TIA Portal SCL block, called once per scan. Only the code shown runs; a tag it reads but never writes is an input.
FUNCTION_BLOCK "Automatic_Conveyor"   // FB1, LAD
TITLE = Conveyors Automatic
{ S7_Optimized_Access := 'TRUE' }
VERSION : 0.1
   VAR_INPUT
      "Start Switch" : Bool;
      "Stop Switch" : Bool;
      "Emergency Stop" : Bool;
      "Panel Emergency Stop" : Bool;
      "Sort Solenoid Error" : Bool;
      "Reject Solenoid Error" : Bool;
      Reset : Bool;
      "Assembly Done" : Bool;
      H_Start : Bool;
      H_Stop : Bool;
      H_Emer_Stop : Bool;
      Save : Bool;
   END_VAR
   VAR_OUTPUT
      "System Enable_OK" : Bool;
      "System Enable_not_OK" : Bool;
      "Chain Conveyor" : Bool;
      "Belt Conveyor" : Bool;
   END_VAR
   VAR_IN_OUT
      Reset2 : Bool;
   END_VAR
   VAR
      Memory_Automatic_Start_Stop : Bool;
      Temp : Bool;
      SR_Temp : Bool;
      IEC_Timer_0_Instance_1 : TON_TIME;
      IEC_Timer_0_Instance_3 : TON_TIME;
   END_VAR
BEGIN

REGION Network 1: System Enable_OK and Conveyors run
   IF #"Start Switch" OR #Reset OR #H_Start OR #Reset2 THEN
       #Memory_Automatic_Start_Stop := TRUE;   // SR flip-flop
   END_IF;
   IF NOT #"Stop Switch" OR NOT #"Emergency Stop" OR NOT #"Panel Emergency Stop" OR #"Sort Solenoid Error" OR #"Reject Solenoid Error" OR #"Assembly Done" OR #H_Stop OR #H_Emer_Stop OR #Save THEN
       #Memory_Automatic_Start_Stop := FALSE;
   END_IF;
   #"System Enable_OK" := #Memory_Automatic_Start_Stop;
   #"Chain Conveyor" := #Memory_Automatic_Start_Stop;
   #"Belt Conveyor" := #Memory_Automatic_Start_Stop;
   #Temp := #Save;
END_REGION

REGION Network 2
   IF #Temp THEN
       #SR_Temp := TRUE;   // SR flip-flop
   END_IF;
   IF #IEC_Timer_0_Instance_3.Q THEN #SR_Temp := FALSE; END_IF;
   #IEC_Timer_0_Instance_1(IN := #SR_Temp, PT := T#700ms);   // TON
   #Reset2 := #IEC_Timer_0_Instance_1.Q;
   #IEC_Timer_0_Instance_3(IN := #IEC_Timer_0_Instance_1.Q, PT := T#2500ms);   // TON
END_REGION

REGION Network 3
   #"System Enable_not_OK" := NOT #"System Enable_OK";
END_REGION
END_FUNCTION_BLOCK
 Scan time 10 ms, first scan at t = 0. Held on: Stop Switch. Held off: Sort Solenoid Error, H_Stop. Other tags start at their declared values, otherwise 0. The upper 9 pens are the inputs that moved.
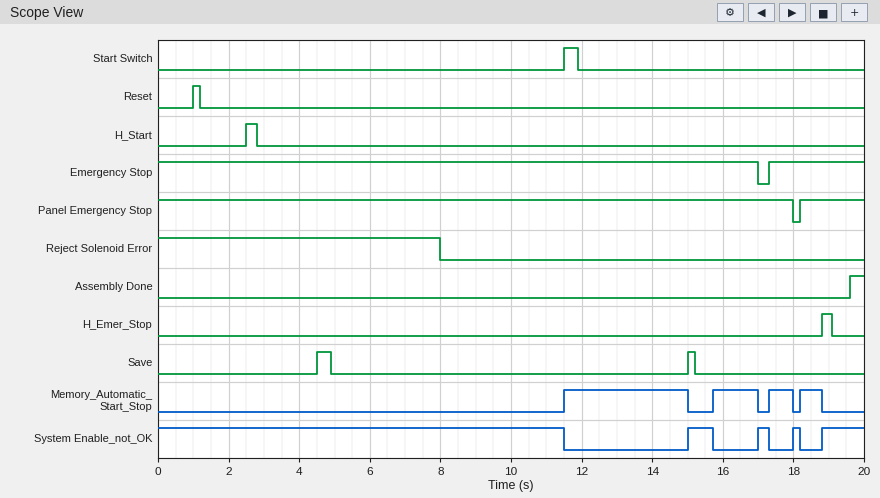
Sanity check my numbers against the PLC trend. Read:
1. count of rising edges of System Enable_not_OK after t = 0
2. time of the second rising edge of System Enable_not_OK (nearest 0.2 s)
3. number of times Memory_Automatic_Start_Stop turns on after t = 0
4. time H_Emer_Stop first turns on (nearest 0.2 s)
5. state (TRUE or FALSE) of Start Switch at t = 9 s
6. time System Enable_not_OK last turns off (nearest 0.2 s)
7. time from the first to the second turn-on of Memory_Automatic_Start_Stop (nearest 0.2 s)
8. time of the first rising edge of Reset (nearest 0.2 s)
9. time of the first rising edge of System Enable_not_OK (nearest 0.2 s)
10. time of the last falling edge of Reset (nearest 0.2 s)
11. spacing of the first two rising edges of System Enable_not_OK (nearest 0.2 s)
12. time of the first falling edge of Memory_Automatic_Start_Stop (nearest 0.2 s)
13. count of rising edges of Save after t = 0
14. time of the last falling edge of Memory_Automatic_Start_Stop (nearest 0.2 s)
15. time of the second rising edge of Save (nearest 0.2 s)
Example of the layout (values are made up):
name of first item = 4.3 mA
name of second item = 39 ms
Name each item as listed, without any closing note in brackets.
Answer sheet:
count of rising edges of System Enable_not_OK after t = 0 = 4
time of the second rising edge of System Enable_not_OK = 17.0 s
number of times Memory_Automatic_Start_Stop turns on after t = 0 = 4
time H_Emer_Stop first turns on = 18.8 s
state (TRUE or FALSE) of Start Switch at t = 9 s = FALSE
time System Enable_not_OK last turns off = 18.2 s
time from the first to the second turn-on of Memory_Automatic_Start_Stop = 4.2 s
time of the first rising edge of Reset = 1.0 s
time of the first rising edge of System Enable_not_OK = 15.0 s
time of the last falling edge of Reset = 1.2 s
spacing of the first two rising edges of System Enable_not_OK = 2.0 s
time of the first falling edge of Memory_Automatic_Start_Stop = 15.0 s
count of rising edges of Save after t = 0 = 2
time of the last falling edge of Memory_Automatic_Start_Stop = 18.8 s
time of the second rising edge of Save = 15.0 s
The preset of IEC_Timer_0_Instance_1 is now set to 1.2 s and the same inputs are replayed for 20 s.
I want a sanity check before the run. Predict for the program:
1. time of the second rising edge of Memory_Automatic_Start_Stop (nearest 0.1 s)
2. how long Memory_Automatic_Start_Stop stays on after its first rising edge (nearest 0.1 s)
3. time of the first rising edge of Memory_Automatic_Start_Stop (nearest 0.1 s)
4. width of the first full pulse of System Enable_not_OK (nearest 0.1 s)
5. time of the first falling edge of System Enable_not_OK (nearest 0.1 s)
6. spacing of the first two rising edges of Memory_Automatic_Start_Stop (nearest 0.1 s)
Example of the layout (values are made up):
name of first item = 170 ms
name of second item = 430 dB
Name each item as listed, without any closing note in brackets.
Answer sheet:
time of the second rising edge of Memory_Automatic_Start_Stop = 16.2 s
how long Memory_Automatic_Start_Stop stays on after its first rising edge = 7.0 s
time of the first rising edge of Memory_Automatic_Start_Stop = 8.0 s
width of the first full pulse of System Enable_not_OK = 1.2 s
time of the first falling edge of System Enable_not_OK = 8.0 s
spacing of the first two rising edges of Memory_Automatic_Start_Stop = 8.2 s
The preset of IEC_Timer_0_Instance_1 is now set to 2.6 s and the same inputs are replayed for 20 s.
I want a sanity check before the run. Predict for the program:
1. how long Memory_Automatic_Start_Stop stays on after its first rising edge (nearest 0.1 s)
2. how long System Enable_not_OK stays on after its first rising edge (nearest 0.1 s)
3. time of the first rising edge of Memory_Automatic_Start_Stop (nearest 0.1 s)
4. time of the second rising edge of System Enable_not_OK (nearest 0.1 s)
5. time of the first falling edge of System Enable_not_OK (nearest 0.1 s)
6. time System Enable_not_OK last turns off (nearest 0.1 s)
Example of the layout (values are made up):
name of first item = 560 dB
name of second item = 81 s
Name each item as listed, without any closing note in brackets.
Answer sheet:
how long Memory_Automatic_Start_Stop stays on after its first rising edge = 7.0 s
how long System Enable_not_OK stays on after its first rising edge = 2.6 s
time of the first rising edge of Memory_Automatic_Start_Stop = 8.0 s
time of the second rising edge of System Enable_not_OK = 18.0 s
time of the first falling edge of System Enable_not_OK = 8.0 s
time System Enable_not_OK last turns off = 19.1 s
